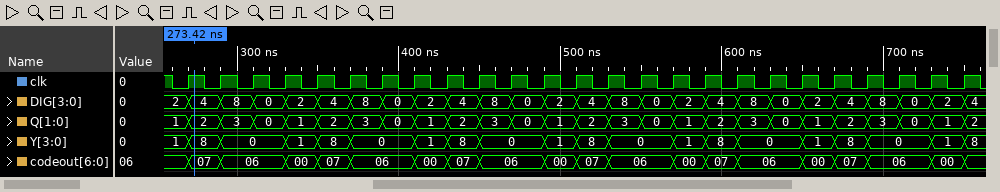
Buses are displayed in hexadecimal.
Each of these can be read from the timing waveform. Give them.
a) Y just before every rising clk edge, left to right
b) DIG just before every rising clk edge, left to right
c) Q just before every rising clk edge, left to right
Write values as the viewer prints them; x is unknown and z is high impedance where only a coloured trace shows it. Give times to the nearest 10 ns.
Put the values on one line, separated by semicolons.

1, 8, 0, 0, 1, 8, 0, 0, 1, 8, 0, 0, 1, 8, 0, 0, 1, 8, 0, 0, 1, 8, 0, 0, 1; 2, 4, 8, 0, 2, 4, 8, 0, 2, 4, 8, 0, 2, 4, 8, 0, 2, 4, 8, 0, 2, 4, 8, 0, 2; 1, 2, 3, 0, 1, 2, 3, 0, 1, 2, 3, 0, 1, 2, 3, 0, 1, 2, 3, 0, 1, 2, 3, 0, 1
